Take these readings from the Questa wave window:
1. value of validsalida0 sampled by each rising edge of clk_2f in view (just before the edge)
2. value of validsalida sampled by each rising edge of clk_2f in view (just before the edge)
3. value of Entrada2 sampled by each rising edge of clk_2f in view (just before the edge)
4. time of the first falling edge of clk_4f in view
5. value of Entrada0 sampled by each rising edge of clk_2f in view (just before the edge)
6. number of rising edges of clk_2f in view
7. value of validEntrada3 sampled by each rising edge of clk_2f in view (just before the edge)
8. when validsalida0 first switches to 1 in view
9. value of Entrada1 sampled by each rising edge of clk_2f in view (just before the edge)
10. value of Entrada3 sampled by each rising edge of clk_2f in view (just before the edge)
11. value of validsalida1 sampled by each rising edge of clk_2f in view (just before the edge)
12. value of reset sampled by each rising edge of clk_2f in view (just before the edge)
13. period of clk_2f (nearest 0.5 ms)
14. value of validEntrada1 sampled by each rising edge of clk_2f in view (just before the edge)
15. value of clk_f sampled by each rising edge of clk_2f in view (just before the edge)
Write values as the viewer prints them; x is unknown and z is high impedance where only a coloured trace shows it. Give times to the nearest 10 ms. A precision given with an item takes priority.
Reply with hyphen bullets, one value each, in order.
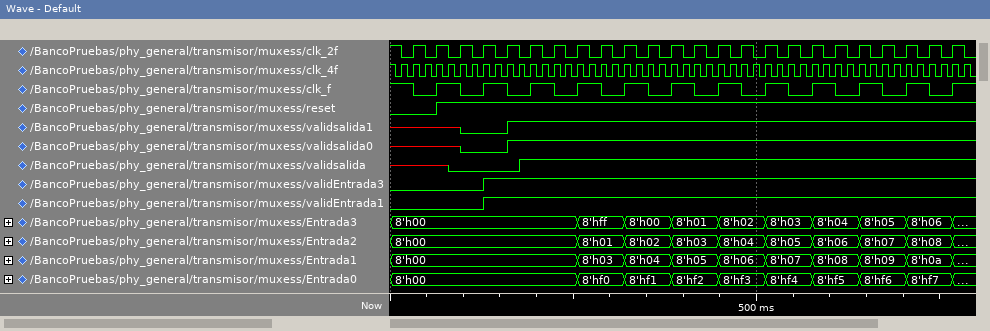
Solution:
- x x x 0 0 1 1 1 1 1 1 1 1 1 1 1 1 1 1 1 1 1 1 1
- x x 0 0 0 1 1 1 1 1 1 1 1 1 1 1 1 1 1 1 1 1 1 1
- 8'h00, 8'h00, 8'h00, 8'h00, 8'h00, 8'h00, 8'h00, 8'h00, 8'h01, 8'h01, 8'h02, 8'h02, 8'h03, 8'h03, 8'h04, 8'h04, 8'h05, 8'h05, 8'h06, 8'h06, 8'h07, 8'h07, 8'h08, 8'h08
- 10 ms
- 8'h00, 8'h00, 8'h00, 8'h00, 8'h00, 8'h00, 8'h00, 8'h00, 8'hf0, 8'hf0, 8'hf1, 8'hf1, 8'hf2, 8'hf2, 8'hf3, 8'hf3, 8'hf4, 8'hf4, 8'hf5, 8'hf5, 8'hf6, 8'hf6, 8'hf7, 8'hf7
- 24
- 0 0 0 0 1 1 1 1 1 1 1 1 1 1 1 1 1 1 1 1 1 1 1 1
- 160 ms
- 8'h00, 8'h00, 8'h00, 8'h00, 8'h00, 8'h00, 8'h00, 8'h00, 8'h03, 8'h03, 8'h04, 8'h04, 8'h05, 8'h05, 8'h06, 8'h06, 8'h07, 8'h07, 8'h08, 8'h08, 8'h09, 8'h09, 8'h0a, 8'h0a
- 8'h00, 8'h00, 8'h00, 8'h00, 8'h00, 8'h00, 8'h00, 8'h00, 8'hff, 8'hff, 8'h00, 8'h00, 8'h01, 8'h01, 8'h02, 8'h02, 8'h03, 8'h03, 8'h04, 8'h04, 8'h05, 8'h05, 8'h06, 8'h06
- x x x 0 0 1 1 1 1 1 1 1 1 1 1 1 1 1 1 1 1 1 1 1
- 0 0 1 1 1 1 1 1 1 1 1 1 1 1 1 1 1 1 1 1 1 1 1 1
- 32 ms
- 0 0 0 0 1 1 1 1 1 1 1 1 1 1 1 1 1 1 1 1 1 1 1 1
- 1 0 1 0 1 0 1 0 1 0 1 0 1 0 1 0 1 0 1 0 1 0 1 0
